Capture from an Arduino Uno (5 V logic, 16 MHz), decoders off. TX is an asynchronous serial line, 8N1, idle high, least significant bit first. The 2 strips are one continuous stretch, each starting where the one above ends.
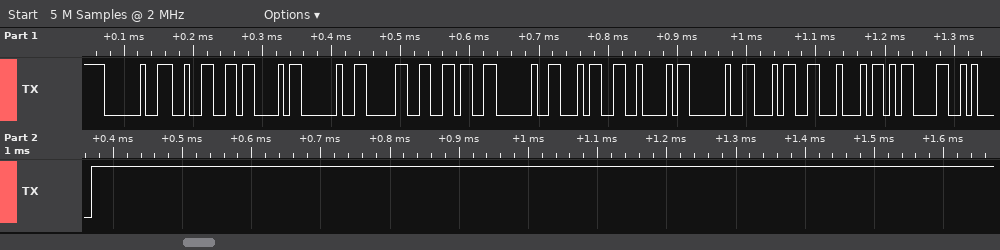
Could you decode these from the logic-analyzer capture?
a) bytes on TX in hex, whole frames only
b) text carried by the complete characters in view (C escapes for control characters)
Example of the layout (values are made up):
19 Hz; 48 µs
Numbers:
0x20 0x32 0x43 0x20 0x30 0x36 0x20 0x34 0x42 0x20 0x34 0x44 0x0D 0x0A; " 2C 06 4B 4D\r\n"
